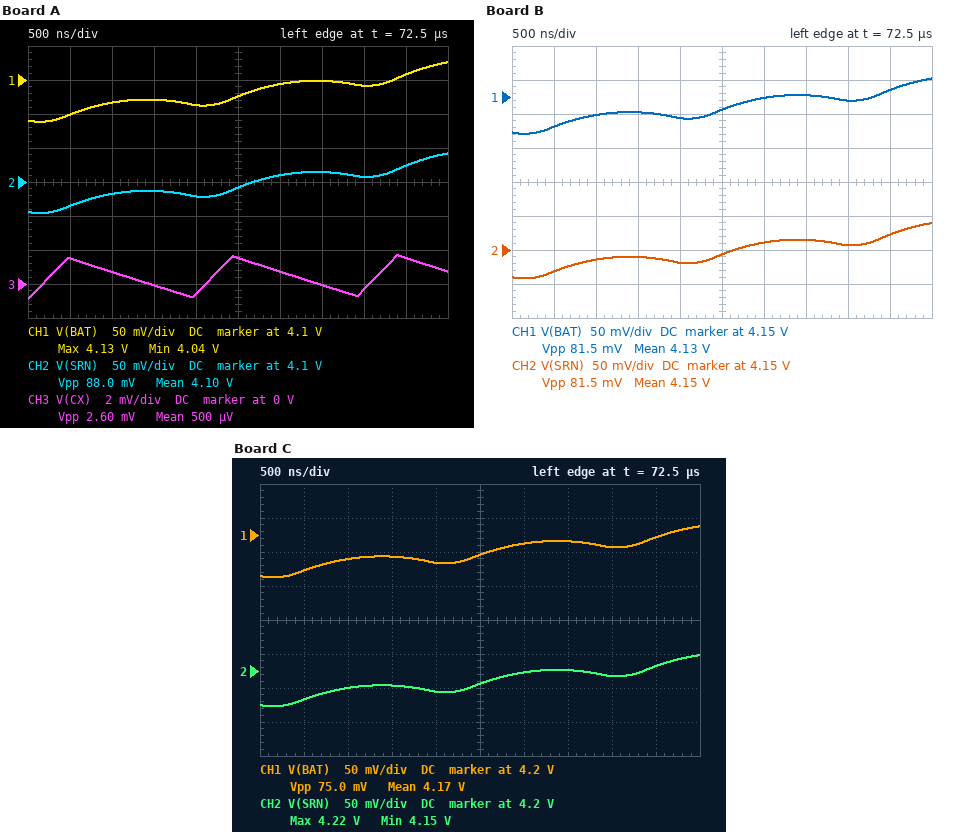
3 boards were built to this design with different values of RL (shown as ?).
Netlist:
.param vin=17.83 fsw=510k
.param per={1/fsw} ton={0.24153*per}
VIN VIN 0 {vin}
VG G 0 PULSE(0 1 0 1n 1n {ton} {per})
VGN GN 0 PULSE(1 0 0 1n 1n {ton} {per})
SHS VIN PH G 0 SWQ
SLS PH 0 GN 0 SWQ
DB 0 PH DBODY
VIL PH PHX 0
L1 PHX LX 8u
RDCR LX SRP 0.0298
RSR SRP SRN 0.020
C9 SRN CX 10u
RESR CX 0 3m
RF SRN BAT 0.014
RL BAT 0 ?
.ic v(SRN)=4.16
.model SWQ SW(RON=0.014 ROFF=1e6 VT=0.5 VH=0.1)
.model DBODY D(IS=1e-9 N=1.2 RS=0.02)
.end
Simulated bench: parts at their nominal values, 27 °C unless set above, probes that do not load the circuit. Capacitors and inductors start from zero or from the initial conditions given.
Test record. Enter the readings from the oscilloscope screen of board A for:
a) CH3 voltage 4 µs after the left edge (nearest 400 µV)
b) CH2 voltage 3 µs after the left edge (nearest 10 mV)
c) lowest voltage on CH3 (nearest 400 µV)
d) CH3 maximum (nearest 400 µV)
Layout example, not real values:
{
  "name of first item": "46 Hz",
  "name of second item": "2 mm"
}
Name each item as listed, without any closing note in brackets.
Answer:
{
  "CH3 voltage 4 µs after the left edge": "-400 µV",
  "CH2 voltage 3 µs after the left edge": "4.11 V",
  "lowest voltage on CH3": "-800 µV",
  "CH3 maximum": "1.6 mV"
}
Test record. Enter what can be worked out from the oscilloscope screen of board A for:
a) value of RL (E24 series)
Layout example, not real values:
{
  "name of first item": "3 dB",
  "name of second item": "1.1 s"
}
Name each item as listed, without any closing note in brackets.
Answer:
{
  "value of RL": "3.6 Ω"
}
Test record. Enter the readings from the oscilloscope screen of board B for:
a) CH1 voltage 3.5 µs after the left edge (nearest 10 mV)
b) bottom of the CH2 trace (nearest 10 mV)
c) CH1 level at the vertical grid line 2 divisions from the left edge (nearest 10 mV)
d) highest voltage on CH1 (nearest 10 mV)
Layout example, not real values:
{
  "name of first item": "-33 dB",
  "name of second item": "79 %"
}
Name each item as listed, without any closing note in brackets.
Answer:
{
  "CH1 voltage 3.5 µs after the left edge": "4.15 V",
  "bottom of the CH2 trace": "4.11 V",
  "CH1 level at the vertical grid line 2 divisions from the left edge": "4.12 V",
  "highest voltage on CH1": "4.18 V"
}
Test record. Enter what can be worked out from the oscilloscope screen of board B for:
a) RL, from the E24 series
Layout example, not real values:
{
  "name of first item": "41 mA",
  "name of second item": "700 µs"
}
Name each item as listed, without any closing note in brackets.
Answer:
{
  "RL, from the E24 series": "4.7 Ω"
}
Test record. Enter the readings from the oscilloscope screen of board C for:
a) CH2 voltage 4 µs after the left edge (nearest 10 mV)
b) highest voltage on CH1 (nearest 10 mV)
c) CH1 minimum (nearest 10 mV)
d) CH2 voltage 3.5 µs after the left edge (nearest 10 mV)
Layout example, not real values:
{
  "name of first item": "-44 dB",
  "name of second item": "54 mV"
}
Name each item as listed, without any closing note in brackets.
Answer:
{
  "CH2 voltage 4 µs after the left edge": "4.19 V",
  "highest voltage on CH1": "4.21 V",
  "CH1 minimum": "4.14 V",
  "CH2 voltage 3.5 µs after the left edge": "4.20 V"
}
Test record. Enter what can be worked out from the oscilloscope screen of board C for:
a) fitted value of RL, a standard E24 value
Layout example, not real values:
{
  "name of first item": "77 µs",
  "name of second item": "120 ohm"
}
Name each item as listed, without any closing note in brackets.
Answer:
{
  "fitted value of RL, a standard E24 value": "5.6 Ω"
}
